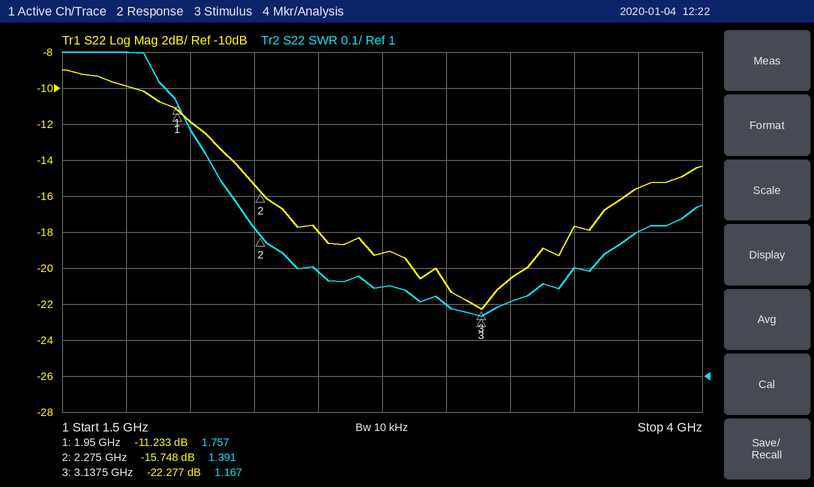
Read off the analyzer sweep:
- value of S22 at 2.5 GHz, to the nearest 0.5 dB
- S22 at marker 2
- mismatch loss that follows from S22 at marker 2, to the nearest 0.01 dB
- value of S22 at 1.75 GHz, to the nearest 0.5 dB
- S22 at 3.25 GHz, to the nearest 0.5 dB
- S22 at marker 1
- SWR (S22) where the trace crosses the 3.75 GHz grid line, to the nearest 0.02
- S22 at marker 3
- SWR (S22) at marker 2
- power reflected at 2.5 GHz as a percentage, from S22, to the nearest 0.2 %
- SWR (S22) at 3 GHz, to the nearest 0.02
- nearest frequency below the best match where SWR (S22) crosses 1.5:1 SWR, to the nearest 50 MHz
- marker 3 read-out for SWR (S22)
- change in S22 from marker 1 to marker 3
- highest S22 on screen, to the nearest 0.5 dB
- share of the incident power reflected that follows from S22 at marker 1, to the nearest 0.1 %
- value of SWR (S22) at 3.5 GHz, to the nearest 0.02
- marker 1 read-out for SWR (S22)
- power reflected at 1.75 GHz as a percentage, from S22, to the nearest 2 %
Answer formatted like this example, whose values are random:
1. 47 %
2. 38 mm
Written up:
1. -18.0 dB
2. -15.748 dB
3. 0.12 dB
4. -10.0 dB
5. -20.5 dB
6. -11.233 dB
7. 1.40
8. -22.277 dB
9. 1.391
10. 1.6 %
11. 1.20
12. 2.15 GHz
13. 1.167
14. -11.044 dB
15. -9.0 dB
16. 7.5 %
17. 1.30
18. 1.757
19. 10 %
